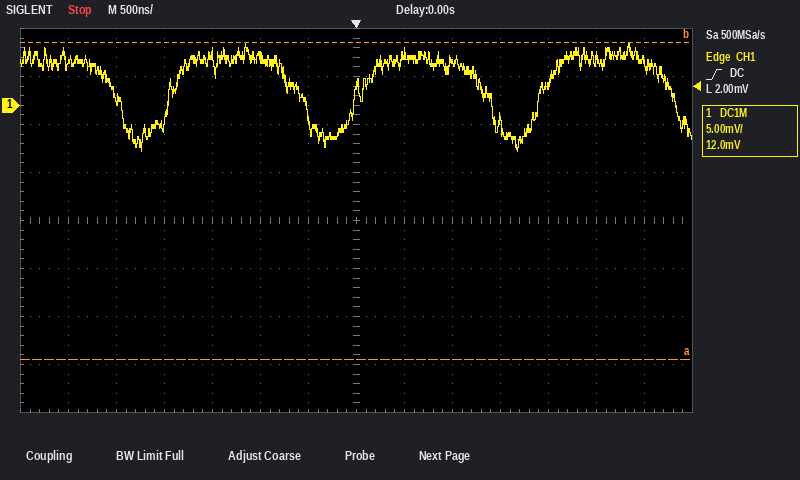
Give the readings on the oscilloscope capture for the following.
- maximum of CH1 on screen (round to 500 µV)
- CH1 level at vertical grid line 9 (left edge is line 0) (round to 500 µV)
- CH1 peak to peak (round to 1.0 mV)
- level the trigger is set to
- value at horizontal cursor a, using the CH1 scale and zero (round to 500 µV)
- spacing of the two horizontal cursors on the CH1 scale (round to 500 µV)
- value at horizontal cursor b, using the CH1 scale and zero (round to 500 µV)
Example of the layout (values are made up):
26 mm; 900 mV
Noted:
6.5 mV; 4.5 mV; 11.0 mV; 2.00 mV; -26.5 mV; 33.0 mV; 6.5 mV
